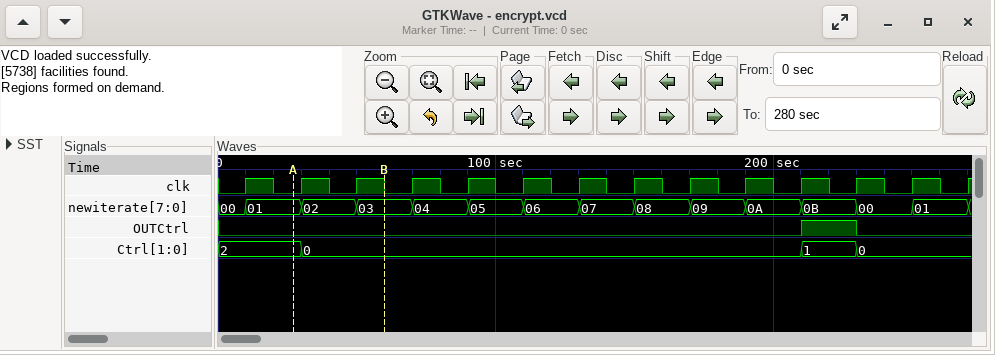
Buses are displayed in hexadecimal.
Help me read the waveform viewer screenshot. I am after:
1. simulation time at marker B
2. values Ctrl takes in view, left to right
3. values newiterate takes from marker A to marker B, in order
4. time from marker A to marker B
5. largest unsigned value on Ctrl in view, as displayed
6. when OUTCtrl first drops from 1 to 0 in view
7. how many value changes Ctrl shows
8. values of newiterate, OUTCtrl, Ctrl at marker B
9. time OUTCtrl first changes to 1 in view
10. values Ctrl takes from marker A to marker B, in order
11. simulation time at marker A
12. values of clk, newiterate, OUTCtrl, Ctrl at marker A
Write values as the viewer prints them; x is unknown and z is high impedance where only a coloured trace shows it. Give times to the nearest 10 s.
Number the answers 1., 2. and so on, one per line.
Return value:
1. 60 s
2. 2, 0, 1, 0
3. 01, 02, 03
4. 30 s
5. 2
6. 230 s
7. 3
8. newiterate=03, OUTCtrl=0, Ctrl=0
9. 210 s
10. 2, 0
11. 30 s
12. clk=0, newiterate=01, OUTCtrl=0, Ctrl=2
